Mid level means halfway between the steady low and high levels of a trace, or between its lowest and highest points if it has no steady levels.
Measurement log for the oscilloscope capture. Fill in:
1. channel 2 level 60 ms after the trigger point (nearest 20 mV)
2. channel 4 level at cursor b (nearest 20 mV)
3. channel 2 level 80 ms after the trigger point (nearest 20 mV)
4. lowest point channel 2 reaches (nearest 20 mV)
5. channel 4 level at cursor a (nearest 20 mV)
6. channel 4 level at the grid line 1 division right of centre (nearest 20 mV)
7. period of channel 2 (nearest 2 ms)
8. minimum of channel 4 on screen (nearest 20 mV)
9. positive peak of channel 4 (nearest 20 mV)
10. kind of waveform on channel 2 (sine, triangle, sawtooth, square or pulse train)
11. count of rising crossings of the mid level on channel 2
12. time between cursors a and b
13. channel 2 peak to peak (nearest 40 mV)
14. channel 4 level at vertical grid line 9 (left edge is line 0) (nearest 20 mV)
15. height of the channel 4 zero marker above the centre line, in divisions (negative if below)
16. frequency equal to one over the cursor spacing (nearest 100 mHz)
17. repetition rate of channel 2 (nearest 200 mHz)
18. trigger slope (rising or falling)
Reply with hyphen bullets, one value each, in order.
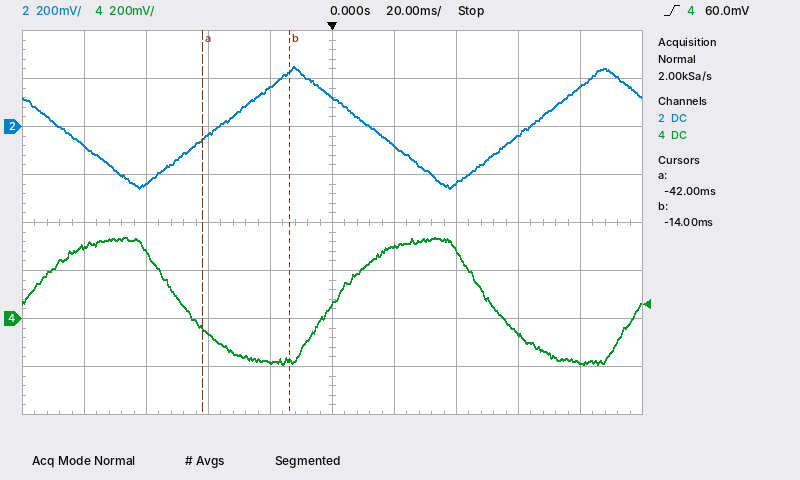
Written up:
- -40 mV
- -180 mV
- 160 mV
- -260 mV
- -40 mV
- 300 mV
- 100 ms
- -200 mV
- 340 mV
- triangle
- 2
- 28 ms
- 520 mV
- -180 mV
- -2.0 div
- 35.7 Hz
- 10.0 Hz
- rising
